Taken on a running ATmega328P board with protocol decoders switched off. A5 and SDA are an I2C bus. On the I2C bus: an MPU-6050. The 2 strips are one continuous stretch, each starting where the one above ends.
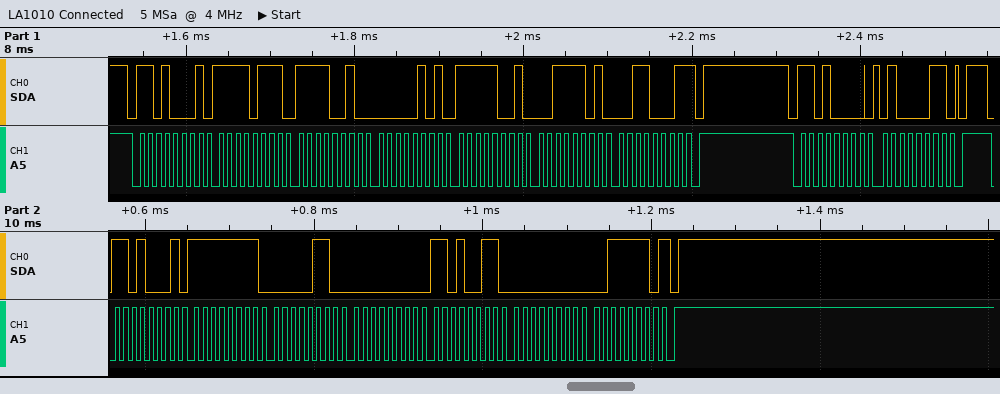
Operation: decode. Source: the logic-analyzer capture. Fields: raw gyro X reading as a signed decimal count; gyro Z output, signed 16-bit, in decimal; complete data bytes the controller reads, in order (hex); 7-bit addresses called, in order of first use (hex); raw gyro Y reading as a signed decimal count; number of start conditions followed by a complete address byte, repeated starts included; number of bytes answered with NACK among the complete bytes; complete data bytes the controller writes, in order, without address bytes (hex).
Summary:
-250
62
F7 F2 05 F9 3D 31 FF 06 00 D3 00 3E
0x68
211
3
2
43
